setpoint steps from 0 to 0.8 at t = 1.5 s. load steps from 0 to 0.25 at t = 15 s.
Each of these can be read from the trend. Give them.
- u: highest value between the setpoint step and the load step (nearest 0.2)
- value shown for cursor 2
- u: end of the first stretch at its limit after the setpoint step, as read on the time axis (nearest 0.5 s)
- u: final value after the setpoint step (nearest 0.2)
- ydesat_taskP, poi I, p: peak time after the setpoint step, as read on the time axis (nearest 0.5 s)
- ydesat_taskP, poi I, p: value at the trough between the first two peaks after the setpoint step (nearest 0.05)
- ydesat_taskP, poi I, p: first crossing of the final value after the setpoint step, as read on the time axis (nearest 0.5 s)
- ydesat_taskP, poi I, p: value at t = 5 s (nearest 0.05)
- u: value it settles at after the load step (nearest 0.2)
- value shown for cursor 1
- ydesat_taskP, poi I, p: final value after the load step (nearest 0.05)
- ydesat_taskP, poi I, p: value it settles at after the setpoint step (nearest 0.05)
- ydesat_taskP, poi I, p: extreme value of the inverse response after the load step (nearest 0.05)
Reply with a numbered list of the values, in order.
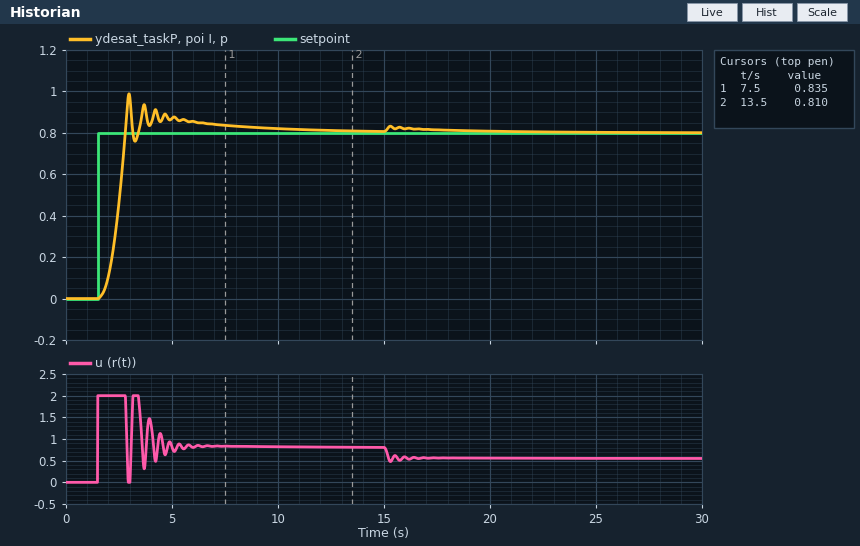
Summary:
1. 2.0
2. 0.810
3. 3.0 s
4. 0.8
5. 3.0 s
6. 0.75
7. 3.0 s
8. 0.85
9. 0.6
10. 0.835
11. 0.80
12. 0.80
13. 0.85
